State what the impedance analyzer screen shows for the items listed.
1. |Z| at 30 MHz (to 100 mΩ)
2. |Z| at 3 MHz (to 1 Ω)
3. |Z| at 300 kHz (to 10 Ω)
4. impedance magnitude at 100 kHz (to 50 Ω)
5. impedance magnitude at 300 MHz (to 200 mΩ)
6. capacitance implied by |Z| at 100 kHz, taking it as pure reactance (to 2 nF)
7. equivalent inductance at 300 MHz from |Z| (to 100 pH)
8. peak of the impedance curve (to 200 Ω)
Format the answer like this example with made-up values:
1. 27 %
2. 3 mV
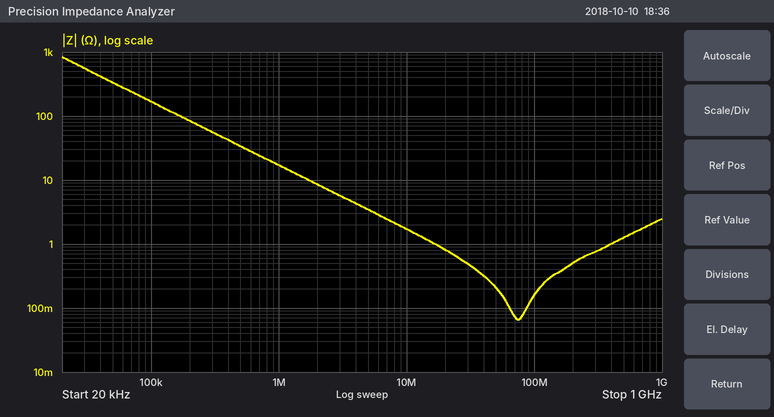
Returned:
1. 500 mΩ
2. 6 Ω
3. 60 Ω
4. 150 Ω
5. 800 mΩ
6. 10 nF
7. 400 pH
8. 800 Ω
